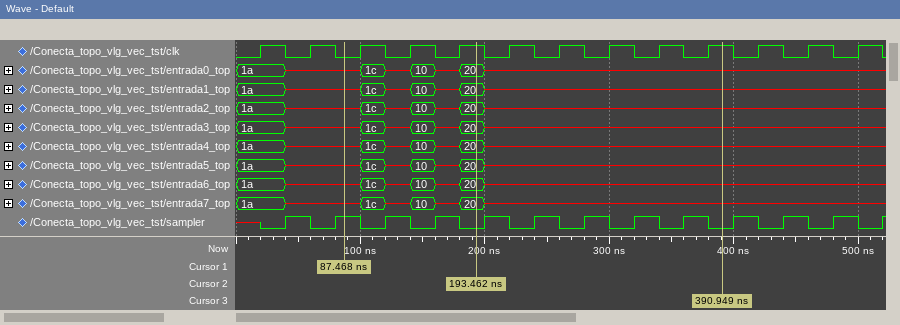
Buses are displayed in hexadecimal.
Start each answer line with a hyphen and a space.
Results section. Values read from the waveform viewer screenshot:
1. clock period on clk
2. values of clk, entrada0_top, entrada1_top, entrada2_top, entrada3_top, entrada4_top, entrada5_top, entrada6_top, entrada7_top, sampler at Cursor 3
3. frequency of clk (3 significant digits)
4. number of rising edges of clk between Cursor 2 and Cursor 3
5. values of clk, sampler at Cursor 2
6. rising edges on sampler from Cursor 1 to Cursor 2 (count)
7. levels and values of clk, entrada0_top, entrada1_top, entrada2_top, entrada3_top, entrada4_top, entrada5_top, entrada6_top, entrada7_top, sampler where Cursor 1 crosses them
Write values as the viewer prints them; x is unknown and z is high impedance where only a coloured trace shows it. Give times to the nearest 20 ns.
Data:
- 40 ns
- clk=1, entrada0_top=x, entrada1_top=x, entrada2_top=x, entrada3_top=x, entrada4_top=x, entrada5_top=x, entrada6_top=x, entrada7_top=x, sampler=0
- 25.0 MHz
- 5
- clk=1, sampler=0
- 2
- clk=0, entrada0_top=x, entrada1_top=x, entrada2_top=x, entrada3_top=x, entrada4_top=x, entrada5_top=x, entrada6_top=x, entrada7_top=x, sampler=1
